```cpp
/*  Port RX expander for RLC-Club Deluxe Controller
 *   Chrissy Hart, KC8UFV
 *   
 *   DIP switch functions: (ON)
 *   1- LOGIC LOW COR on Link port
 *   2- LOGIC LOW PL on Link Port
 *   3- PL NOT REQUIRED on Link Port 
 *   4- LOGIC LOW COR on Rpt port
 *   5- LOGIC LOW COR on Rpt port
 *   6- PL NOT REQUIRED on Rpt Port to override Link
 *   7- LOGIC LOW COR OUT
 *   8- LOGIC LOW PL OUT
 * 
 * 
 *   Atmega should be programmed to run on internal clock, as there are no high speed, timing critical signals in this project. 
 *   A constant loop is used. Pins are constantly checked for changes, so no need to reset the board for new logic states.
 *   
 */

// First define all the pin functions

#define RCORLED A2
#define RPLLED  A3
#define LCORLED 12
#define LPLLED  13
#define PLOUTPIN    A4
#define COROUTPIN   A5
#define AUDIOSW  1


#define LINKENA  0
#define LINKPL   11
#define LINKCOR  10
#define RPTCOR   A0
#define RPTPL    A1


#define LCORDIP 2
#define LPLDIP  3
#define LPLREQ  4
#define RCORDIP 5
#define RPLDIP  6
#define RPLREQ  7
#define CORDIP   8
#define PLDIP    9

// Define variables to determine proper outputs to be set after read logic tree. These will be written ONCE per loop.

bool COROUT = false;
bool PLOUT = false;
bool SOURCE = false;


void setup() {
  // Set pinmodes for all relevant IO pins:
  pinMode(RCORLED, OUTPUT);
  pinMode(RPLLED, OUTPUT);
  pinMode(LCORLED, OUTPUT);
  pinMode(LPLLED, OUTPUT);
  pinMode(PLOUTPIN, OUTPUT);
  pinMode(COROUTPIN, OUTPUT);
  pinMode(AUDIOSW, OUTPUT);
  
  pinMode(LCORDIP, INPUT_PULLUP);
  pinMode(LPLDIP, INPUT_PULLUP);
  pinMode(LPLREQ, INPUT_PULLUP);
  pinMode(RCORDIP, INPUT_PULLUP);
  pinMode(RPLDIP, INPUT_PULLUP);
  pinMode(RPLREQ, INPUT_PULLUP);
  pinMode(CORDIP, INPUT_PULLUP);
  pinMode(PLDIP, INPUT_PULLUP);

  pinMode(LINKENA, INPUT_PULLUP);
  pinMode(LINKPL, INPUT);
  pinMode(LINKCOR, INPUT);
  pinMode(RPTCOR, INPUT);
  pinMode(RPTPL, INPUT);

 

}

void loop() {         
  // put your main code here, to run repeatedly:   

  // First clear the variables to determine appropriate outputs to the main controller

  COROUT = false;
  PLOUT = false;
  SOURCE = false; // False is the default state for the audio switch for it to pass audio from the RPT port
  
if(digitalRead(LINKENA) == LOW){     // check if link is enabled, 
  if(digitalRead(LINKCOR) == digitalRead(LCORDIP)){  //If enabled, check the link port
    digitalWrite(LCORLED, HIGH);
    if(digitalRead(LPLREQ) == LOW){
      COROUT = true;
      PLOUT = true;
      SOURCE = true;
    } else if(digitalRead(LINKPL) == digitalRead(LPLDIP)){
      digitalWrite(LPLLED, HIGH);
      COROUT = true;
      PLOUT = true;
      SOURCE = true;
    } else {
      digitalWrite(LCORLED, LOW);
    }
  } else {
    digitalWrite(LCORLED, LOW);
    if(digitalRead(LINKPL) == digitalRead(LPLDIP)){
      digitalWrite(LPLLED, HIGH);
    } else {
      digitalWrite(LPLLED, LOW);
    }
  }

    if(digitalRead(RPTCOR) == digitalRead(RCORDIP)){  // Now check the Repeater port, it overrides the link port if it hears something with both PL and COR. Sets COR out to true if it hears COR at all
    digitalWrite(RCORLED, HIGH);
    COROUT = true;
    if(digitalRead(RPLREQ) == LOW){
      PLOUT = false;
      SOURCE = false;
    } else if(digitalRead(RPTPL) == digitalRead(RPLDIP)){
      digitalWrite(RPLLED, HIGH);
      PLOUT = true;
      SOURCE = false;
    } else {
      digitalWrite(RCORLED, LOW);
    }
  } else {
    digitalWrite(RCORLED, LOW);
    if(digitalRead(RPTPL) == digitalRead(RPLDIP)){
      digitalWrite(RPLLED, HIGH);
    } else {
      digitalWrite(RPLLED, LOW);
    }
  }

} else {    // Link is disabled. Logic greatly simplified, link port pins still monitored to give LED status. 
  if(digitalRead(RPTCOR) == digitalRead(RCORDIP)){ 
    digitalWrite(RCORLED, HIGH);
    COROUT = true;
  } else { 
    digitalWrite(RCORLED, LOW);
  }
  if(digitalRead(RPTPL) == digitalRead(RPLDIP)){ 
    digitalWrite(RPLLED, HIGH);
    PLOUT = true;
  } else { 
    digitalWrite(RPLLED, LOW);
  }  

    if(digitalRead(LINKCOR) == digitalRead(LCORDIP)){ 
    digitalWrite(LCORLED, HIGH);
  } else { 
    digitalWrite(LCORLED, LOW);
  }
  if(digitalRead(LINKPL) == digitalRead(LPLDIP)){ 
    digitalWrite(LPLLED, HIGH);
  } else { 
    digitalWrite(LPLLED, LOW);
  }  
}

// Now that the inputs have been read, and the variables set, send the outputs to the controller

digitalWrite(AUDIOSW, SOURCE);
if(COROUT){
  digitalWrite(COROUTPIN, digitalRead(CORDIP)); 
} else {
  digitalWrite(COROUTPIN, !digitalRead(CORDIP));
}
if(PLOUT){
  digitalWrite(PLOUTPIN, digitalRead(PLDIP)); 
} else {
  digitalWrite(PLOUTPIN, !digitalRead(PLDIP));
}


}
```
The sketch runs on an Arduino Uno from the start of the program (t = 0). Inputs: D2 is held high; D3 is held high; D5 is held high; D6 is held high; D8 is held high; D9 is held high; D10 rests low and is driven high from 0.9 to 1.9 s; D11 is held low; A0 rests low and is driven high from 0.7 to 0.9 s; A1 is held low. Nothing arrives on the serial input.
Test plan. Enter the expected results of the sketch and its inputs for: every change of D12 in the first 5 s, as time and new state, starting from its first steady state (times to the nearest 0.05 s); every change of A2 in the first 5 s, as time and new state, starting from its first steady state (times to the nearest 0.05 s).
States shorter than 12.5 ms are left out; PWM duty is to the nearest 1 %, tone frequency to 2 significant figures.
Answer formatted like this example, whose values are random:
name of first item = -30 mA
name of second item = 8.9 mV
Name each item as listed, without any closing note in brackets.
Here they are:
every change of D12 in the first 5 s, as time and new state, starting from its first steady state = 0 s low; 0.9 s high; 1.9 s low
every change of A2 in the first 5 s, as time and new state, starting from its first steady state = 0 s low; 0.7 s high; 0.9 s low
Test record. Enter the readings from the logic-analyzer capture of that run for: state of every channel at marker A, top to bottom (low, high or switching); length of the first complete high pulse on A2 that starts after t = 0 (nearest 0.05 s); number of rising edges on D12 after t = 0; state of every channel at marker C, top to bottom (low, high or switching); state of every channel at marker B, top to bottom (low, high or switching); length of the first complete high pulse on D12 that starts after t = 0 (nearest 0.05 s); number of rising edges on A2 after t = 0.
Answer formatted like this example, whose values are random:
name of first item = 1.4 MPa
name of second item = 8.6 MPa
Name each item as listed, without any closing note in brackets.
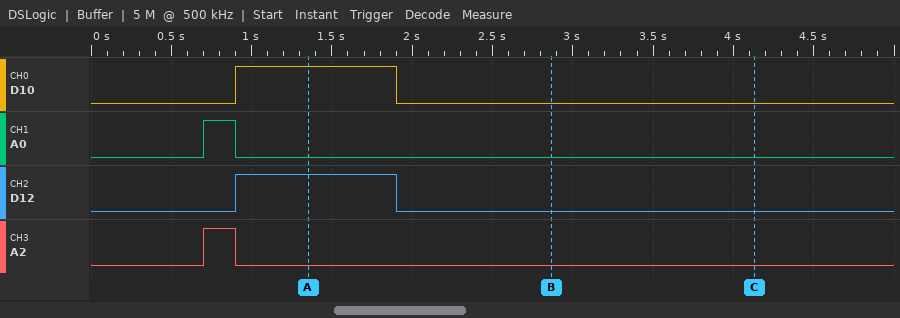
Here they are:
state of every channel at marker A, top to bottom = D10 high, A0 low, D12 high, A2 low
length of the first complete high pulse on A2 that starts after t = 0 = 0.20 s
number of rising edges on D12 after t = 0 = 1
state of every channel at marker C, top to bottom = D10 low, A0 low, D12 low, A2 low
state of every channel at marker B, top to bottom = D10 low, A0 low, D12 low, A2 low
length of the first complete high pulse on D12 that starts after t = 0 = 1.00 s
number of rising edges on A2 after t = 0 = 1
